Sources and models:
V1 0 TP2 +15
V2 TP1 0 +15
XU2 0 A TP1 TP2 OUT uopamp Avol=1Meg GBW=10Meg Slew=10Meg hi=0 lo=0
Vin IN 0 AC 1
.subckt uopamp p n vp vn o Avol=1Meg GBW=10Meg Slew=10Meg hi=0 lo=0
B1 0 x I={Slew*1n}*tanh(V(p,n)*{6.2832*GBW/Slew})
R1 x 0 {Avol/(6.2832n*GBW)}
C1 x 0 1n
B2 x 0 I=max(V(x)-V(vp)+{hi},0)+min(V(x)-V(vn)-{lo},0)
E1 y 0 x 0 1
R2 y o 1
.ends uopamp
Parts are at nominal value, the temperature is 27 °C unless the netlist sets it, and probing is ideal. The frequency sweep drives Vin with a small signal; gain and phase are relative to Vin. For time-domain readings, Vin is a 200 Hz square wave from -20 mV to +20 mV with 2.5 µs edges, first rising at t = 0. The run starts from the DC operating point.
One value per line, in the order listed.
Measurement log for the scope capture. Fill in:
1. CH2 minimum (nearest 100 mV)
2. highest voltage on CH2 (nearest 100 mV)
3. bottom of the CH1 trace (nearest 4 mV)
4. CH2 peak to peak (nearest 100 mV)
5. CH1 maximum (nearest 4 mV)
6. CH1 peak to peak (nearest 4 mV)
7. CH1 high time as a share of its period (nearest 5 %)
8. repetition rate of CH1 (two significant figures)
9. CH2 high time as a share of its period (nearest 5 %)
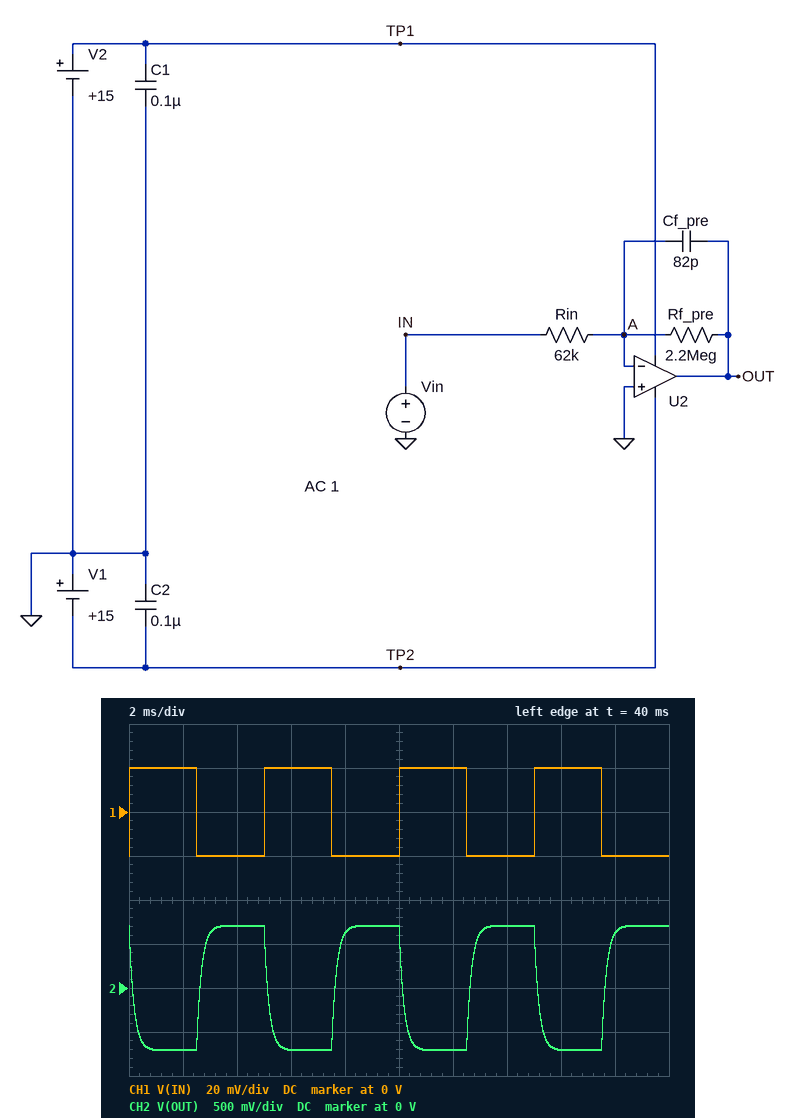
-700 mV
700 mV
-20 mV
1.4 V
20 mV
40 mV
50 %
200 Hz
50 %
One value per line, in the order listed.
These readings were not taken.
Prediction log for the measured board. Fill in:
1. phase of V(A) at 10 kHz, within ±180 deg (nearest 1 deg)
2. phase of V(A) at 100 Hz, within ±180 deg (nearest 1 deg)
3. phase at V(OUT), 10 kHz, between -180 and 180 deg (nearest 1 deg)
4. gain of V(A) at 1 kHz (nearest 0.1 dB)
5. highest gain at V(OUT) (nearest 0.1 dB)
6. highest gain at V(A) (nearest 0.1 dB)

5 deg
78 deg
95 deg
-52.6 dB
31.0 dB
-50.1 dB
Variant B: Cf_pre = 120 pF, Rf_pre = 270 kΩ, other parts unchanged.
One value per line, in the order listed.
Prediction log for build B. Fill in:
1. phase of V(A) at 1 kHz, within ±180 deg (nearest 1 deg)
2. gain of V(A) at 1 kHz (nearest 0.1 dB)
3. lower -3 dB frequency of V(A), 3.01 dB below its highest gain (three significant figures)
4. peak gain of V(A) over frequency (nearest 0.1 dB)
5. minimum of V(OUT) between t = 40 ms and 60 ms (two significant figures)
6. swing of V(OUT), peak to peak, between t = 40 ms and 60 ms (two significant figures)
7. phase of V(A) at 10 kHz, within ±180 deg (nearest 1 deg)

78 deg
-67.4 dB
4.90 kHz
-53.4 dB
-87 mV
170 mV
26 deg
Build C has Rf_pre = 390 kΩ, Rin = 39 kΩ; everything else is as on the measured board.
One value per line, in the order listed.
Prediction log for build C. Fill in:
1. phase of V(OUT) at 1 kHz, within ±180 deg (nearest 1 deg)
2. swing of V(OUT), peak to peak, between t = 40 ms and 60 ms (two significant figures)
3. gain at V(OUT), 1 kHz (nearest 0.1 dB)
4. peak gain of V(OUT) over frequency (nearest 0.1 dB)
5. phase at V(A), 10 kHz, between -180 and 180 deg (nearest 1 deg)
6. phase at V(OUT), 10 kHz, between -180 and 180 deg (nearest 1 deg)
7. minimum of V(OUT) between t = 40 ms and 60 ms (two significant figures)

169 deg
400 mV
19.8 dB
20.0 dB
26 deg
116 deg
-200 mV
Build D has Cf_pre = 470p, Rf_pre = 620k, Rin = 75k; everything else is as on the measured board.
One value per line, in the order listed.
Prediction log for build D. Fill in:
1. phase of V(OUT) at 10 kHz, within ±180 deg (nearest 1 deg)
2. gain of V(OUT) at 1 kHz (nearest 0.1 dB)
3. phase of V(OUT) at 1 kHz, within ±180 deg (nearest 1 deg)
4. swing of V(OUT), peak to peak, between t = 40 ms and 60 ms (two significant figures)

93 deg
12.0 dB
119 deg
330 mV
